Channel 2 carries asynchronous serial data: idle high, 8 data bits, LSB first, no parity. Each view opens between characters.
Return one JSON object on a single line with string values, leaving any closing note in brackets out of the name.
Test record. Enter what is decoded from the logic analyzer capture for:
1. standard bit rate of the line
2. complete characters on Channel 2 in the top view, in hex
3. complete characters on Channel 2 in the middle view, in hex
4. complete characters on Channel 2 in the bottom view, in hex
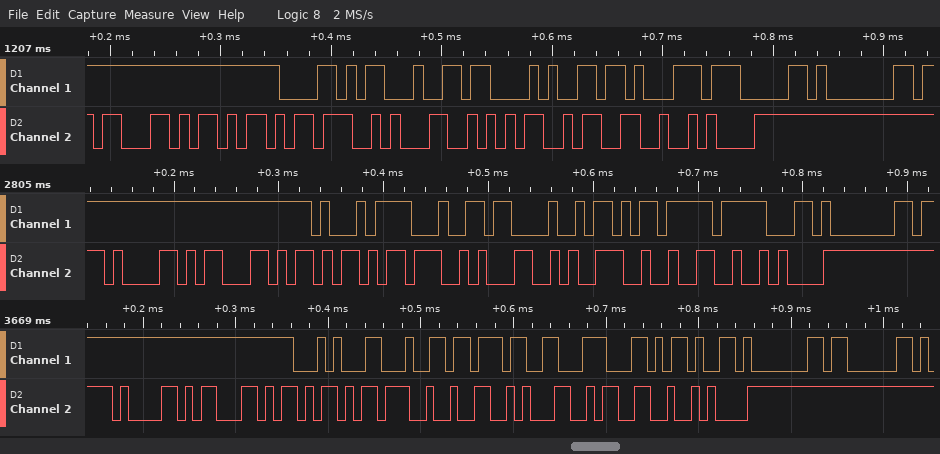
{"standard bit rate of the line": "115200 baud", "complete characters on Channel 2 in the top view, in hex": "63, 6B, 3B, 31, 35, 33, 0A", "complete characters on Channel 2 in the middle view, in hex": "61, 63, 6B, 3B, 31, 39, 32, 0A", "complete characters on Channel 2 in the bottom view, in hex": "61, 63, 6B, 3B, 32, 31, 33, 0A"}
